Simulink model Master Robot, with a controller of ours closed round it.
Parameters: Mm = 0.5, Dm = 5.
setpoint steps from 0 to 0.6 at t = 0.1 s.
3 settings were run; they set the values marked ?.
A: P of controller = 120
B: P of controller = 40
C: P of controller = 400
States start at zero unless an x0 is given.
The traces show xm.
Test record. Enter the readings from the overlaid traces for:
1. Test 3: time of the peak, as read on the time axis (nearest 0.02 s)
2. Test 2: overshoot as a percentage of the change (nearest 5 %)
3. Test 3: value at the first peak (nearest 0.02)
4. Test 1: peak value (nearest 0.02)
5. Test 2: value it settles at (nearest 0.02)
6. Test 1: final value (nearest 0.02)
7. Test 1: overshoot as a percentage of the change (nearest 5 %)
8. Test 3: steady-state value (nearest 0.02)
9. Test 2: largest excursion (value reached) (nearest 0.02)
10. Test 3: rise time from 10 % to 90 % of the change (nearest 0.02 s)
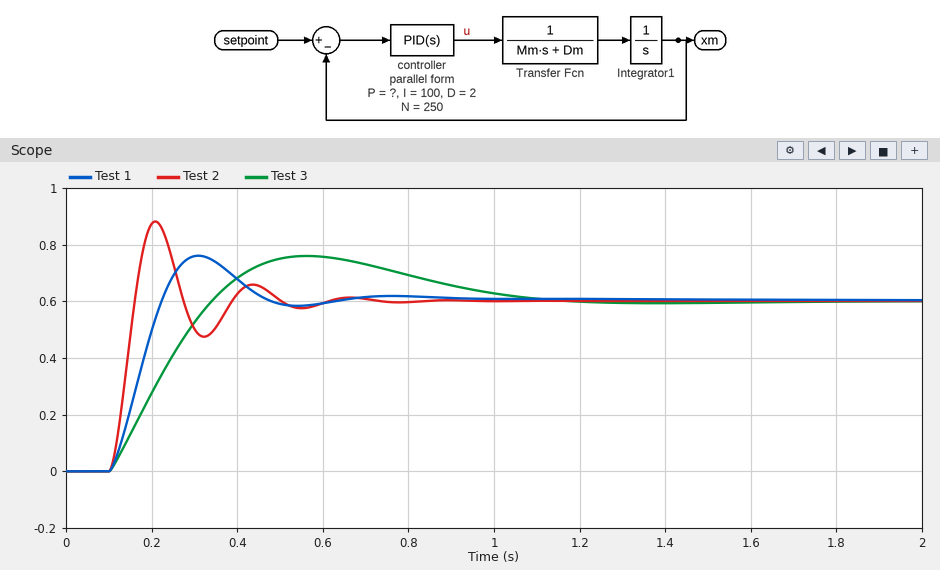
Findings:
0.56 s
45 %
0.76
0.76
0.60
0.60
25 %
0.60
0.88
0.18 s
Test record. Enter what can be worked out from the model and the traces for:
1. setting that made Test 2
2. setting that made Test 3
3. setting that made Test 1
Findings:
C
B
A
